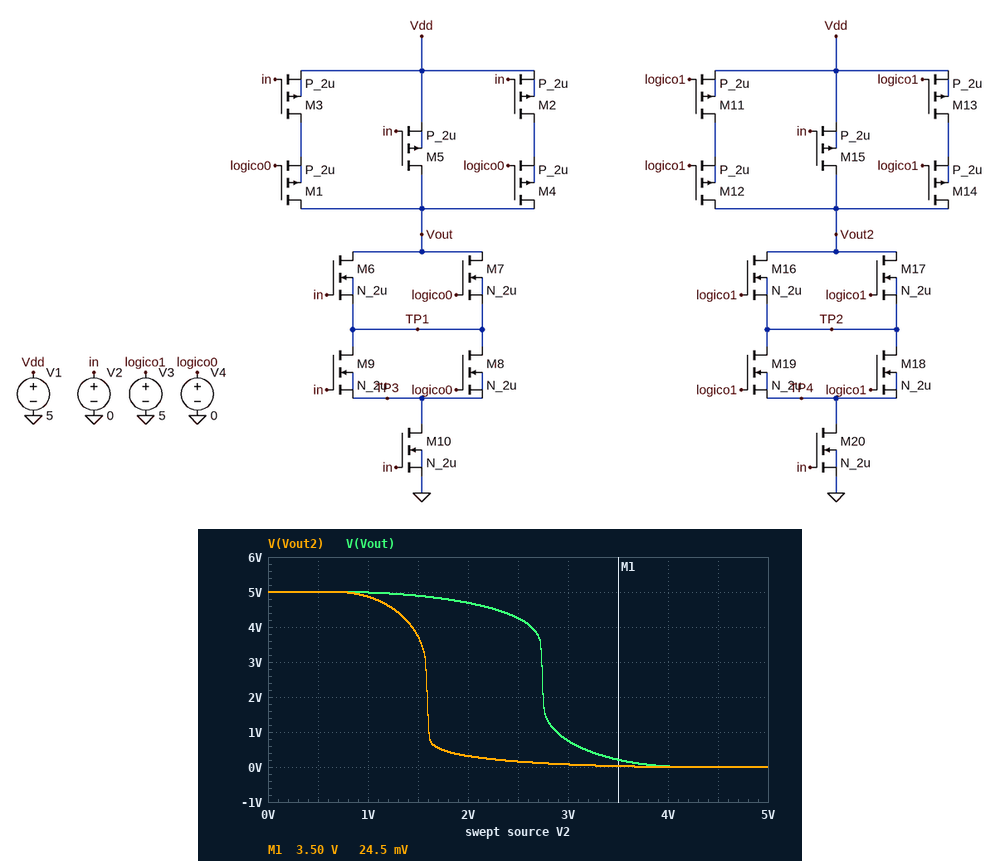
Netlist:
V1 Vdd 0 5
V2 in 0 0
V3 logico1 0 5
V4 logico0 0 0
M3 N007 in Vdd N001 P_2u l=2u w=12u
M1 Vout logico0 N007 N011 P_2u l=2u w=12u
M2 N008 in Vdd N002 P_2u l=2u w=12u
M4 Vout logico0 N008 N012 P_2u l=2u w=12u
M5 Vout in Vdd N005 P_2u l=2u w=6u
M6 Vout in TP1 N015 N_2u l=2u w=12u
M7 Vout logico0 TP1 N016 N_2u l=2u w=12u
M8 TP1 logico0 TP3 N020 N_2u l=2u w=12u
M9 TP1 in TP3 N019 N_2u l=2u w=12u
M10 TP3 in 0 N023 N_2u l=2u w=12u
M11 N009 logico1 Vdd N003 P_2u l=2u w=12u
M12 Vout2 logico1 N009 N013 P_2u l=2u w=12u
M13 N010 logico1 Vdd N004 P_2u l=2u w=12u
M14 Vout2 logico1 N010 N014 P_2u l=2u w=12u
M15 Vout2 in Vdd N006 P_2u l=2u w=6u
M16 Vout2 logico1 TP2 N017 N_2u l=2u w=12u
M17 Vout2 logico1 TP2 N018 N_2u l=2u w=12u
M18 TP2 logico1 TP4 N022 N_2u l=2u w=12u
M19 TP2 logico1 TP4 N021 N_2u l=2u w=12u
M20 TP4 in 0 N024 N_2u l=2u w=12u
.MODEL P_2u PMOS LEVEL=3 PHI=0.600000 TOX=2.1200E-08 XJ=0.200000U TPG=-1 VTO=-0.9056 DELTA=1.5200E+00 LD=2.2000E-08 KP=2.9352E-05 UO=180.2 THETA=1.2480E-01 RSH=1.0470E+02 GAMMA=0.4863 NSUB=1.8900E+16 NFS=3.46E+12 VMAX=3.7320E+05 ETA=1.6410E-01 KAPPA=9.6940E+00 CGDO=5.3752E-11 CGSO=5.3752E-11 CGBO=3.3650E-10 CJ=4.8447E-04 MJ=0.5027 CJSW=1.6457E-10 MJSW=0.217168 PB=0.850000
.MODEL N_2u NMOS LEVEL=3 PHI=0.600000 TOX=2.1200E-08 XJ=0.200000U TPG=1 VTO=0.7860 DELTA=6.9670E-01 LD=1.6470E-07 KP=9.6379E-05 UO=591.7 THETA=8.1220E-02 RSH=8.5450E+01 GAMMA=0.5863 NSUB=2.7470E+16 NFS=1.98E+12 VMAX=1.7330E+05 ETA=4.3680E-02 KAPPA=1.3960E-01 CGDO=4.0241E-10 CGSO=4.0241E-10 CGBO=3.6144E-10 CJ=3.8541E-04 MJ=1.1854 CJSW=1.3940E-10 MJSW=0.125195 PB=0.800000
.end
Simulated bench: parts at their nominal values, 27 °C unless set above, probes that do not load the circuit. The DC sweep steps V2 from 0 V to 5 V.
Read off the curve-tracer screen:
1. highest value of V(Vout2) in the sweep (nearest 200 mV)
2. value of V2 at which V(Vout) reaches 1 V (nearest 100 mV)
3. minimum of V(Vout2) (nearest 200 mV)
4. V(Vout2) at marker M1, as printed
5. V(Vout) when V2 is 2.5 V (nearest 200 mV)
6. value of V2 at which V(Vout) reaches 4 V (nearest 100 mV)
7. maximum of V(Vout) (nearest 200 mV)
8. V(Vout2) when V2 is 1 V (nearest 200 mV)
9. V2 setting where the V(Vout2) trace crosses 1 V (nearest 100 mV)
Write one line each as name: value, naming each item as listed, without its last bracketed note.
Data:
highest value of V(Vout2) in the sweep: 5.0 V
value of V2 at which V(Vout) reaches 1 V: 2.9 V
minimum of V(Vout2): 0 V
V(Vout2) at marker M1, as printed: 24.5 mV
V(Vout) when V2 is 2.5 V: 4.2 V
value of V2 at which V(Vout) reaches 4 V: 2.6 V
maximum of V(Vout): 5.0 V
V(Vout2) when V2 is 1 V: 4.8 V
V2 setting where the V(Vout2) trace crosses 1 V: 1.6 V
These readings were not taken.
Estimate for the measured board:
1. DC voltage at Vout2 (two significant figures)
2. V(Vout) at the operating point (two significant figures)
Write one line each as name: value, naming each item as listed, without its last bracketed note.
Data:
DC voltage at Vout2: 5.0 V
V(Vout) at the operating point: 5.0 V
